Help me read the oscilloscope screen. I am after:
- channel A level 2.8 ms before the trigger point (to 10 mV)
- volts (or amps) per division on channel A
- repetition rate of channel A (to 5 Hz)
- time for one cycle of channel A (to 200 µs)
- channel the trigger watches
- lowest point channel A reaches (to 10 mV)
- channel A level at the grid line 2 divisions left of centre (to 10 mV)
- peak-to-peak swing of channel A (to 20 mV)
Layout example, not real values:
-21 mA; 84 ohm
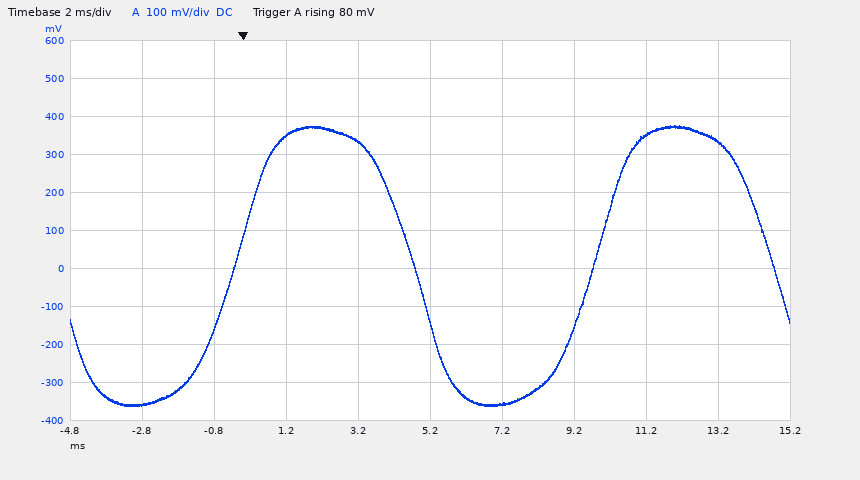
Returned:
-360 mV; 100 mV; 100 Hz; 10.0 ms; channel A; -360 mV; 350 mV; 740 mV
